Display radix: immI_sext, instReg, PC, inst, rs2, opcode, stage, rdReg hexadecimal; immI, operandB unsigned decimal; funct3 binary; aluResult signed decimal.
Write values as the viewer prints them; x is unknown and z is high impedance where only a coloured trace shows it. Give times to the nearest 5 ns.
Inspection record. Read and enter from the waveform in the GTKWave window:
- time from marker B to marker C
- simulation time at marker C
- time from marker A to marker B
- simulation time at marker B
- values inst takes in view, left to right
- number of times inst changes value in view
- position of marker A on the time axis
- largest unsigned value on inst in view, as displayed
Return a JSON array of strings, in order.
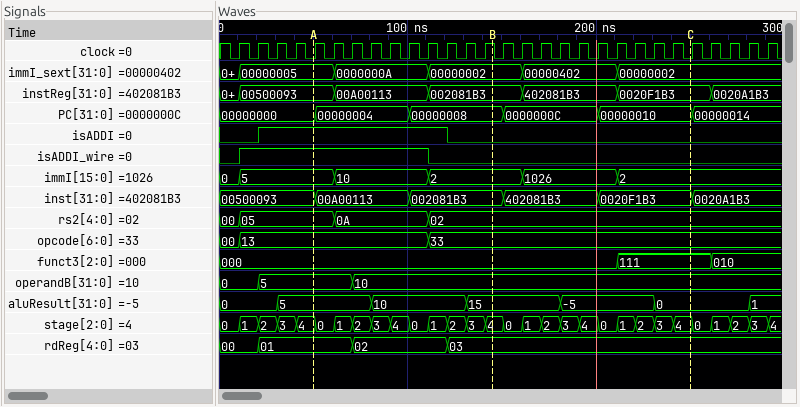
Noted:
["105 ns", "250 ns", "95 ns", "145 ns", "00500093, 00A00113, 002081B3, 402081B3, 0020F1B3, 0020A1B3", "5", "50 ns", "402081B3"]
